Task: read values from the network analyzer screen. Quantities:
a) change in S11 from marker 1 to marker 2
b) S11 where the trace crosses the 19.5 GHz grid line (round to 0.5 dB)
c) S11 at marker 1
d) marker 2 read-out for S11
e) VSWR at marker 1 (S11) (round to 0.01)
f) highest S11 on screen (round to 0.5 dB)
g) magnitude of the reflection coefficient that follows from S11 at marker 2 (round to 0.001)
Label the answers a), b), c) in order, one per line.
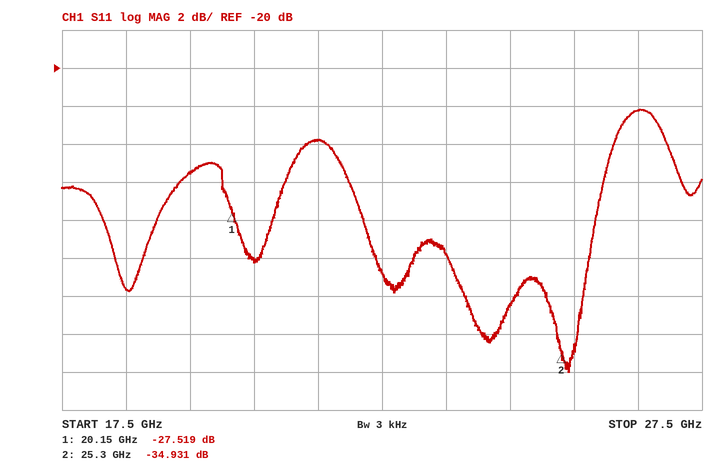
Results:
a) -7.412 dB
b) -25.5 dB
c) -27.519 dB
d) -34.931 dB
e) 1.09
f) -22.0 dB
g) 0.018
